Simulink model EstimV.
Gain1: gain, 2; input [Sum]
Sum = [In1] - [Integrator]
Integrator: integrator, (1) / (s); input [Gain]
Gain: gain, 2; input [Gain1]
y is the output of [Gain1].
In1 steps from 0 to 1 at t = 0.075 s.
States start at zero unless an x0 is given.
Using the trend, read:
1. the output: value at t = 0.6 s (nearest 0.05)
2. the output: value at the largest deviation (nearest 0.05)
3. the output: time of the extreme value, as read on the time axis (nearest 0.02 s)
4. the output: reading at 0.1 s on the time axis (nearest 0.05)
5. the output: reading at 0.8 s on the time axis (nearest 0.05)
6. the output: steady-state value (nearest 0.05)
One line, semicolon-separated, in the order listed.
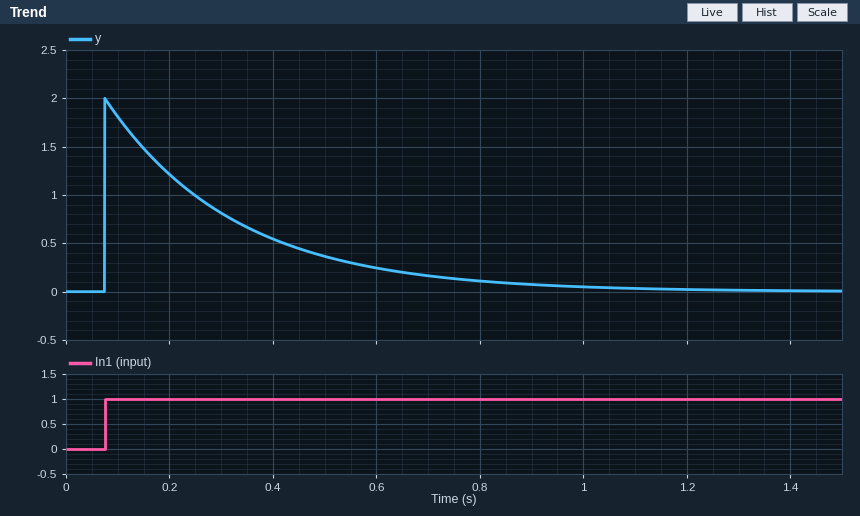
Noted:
0.25; 2.00; 0.08 s; 1.80; 0.10; 0.00
